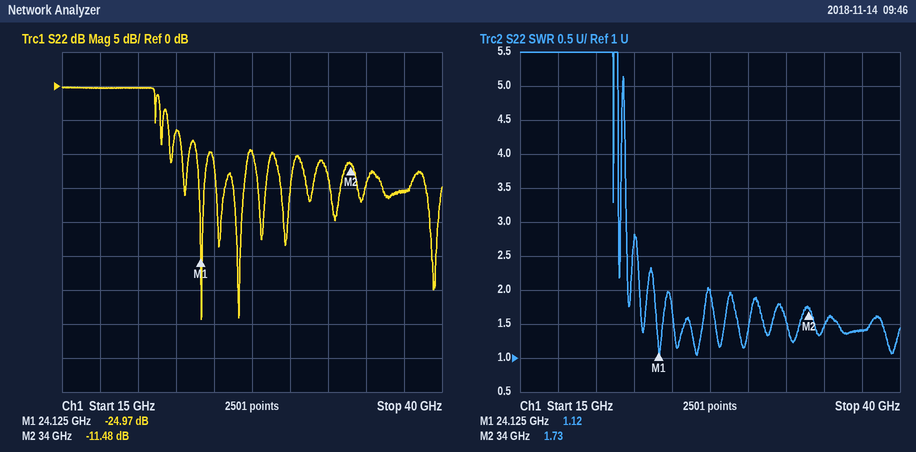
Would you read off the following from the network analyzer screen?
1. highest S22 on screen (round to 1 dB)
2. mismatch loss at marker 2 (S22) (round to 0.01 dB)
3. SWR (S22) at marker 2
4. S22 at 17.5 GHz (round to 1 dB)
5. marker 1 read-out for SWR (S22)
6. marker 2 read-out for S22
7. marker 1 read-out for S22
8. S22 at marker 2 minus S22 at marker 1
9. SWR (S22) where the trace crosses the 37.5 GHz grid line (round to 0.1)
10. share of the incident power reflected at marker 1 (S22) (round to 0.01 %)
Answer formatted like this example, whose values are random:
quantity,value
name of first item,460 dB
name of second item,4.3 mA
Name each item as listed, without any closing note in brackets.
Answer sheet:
quantity,value
highest S22 on screen,0 dB
mismatch loss at marker 2 (S22),0.32 dB
SWR (S22) at marker 2,1.73
S22 at 17.5 GHz,0 dB
marker 1 read-out for SWR,1.12
marker 2 read-out for S22,-11.48 dB
marker 1 read-out for S22,-24.97 dB
S22 at marker 2 minus S22 at marker 1,13.49 dB
SWR (S22) where the trace crosses the 37.5 GHz grid line,1.4
share of the incident power reflected at marker 1 (S22),0.32 %
